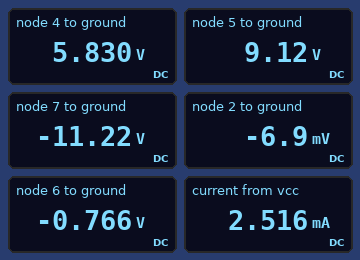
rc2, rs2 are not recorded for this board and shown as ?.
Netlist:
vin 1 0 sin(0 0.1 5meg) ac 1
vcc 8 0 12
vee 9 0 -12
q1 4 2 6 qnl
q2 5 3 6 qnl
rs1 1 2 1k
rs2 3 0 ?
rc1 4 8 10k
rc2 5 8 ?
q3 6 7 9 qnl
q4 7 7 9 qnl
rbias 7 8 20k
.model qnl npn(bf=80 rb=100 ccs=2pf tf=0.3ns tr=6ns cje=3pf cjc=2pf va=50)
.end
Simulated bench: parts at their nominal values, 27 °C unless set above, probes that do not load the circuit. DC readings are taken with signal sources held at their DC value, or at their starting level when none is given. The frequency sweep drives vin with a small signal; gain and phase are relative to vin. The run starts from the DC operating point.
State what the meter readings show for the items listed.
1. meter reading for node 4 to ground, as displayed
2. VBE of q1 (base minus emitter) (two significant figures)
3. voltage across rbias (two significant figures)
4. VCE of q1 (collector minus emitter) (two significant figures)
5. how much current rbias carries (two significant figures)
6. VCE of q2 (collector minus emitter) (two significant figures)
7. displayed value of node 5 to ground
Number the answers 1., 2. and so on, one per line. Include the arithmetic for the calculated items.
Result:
1. 5.830 V
2. -6.9 mV - (-766 mV) = 760 mV
3. 12 V - (-11.22 V) = 23 V
4. 5.83 V - (-766 mV) = 6.6 V
5. (12 V - (-11.22 V)) / 20 kΩ = 1.2 mA
6. 9.12 V - (-766 mV) = 9.9 V
7. 9.12 V
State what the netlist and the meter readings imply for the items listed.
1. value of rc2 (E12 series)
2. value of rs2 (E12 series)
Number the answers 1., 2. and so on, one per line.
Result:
1. 3.9 kΩ
2. 470 Ω
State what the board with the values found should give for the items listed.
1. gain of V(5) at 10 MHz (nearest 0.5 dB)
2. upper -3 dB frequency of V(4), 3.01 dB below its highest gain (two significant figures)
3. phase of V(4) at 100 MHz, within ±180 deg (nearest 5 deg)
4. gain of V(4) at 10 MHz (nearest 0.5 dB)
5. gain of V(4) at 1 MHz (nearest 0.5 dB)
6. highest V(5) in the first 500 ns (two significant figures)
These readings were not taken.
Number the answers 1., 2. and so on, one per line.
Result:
1. 16.0 dB
2. 1.0 MHz
3. 45 deg
4. 19.0 dB
5. 37.0 dB
6. 10 V
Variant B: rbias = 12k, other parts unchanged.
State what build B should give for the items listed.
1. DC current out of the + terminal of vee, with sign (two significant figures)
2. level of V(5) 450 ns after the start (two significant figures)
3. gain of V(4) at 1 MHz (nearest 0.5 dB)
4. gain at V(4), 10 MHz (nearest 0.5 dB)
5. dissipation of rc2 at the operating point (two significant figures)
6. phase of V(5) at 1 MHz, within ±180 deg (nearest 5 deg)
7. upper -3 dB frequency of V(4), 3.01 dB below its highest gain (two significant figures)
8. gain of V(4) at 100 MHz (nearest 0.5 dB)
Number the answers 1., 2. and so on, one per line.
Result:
1. -4.2 mA
2. 7.5 V
3. 37.0 dB
4. 18.0 dB
5. 6.4 mW
6. -50 deg
7. 650 kHz
8. -4.0 dB
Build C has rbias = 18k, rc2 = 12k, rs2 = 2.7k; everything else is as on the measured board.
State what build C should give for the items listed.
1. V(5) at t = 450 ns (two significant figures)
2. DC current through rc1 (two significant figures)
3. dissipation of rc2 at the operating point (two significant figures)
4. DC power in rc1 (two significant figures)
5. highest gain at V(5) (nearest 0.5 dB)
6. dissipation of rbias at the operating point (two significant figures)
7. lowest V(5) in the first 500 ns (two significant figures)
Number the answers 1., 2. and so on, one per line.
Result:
1. 4.7 V
2. 870 µA
3. 4.8 mW
4. 7.6 mW
5. 39.0 dB
6. 30 mW
7. 4.0 V
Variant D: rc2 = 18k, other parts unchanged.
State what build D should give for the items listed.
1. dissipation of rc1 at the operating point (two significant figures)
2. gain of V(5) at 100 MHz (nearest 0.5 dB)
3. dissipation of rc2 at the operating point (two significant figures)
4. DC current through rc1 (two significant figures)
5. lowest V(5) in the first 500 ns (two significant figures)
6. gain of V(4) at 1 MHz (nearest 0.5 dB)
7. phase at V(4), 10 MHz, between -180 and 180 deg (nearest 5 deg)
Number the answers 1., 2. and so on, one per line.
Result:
1. 4.5 mW
2. -11.5 dB
3. 8.4 mW
4. 670 µA
5. -730 mV
6. 31.5 dB
7. 100 deg
